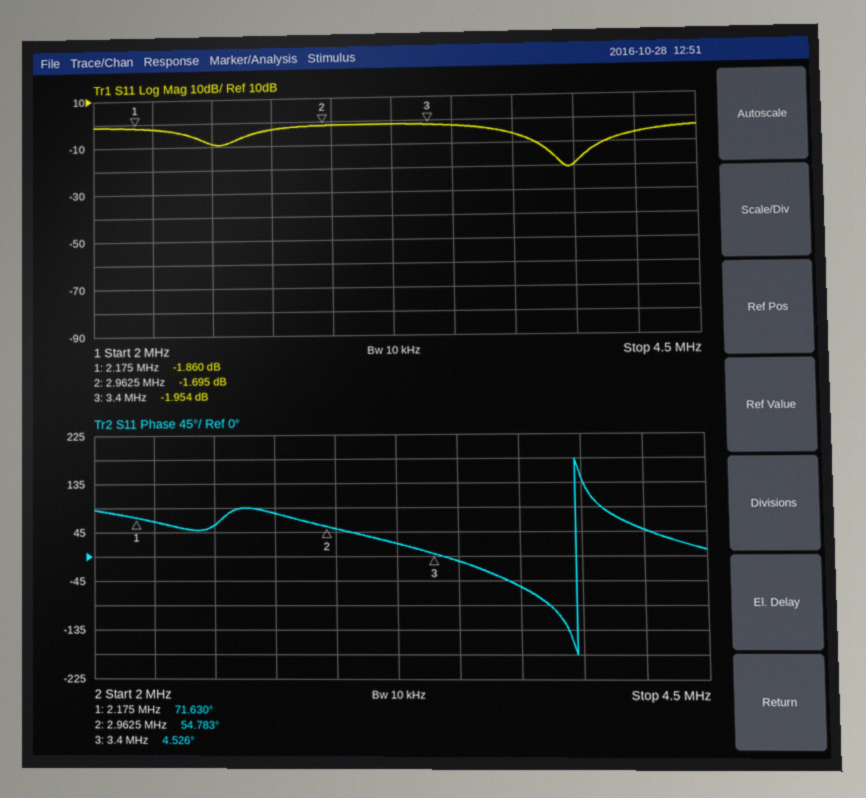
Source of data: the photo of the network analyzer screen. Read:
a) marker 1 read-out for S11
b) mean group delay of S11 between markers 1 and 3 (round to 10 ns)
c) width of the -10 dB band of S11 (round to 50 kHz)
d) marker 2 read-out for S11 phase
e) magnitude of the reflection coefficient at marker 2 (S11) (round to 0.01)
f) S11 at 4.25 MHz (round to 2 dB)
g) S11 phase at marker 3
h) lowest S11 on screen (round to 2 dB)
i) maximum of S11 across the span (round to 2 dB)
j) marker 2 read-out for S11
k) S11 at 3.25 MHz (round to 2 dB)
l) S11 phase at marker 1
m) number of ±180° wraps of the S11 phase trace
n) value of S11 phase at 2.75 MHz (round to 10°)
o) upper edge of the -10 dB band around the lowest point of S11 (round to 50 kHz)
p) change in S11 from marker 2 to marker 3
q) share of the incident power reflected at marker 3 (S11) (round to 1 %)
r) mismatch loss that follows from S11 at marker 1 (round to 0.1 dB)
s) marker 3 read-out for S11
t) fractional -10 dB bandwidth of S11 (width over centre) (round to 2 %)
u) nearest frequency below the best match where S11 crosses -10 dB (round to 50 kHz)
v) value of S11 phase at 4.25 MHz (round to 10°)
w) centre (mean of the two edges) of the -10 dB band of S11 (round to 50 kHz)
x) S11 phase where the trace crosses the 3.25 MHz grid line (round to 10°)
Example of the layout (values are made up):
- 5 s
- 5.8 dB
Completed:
- -1.860 dB
- 150 ns
- 300 kHz
- 54.783°
- 0.82
- -6 dB
- 4.526°
- -20 dB
- -2 dB
- -1.695 dB
- -2 dB
- 71.630°
- 1
- 80°
- 4.15 MHz
- -0.259 dB
- 64 %
- 4.6 dB
- -1.954 dB
- 8 %
- 3.85 MHz
- 50°
- 4.00 MHz
- 20°
